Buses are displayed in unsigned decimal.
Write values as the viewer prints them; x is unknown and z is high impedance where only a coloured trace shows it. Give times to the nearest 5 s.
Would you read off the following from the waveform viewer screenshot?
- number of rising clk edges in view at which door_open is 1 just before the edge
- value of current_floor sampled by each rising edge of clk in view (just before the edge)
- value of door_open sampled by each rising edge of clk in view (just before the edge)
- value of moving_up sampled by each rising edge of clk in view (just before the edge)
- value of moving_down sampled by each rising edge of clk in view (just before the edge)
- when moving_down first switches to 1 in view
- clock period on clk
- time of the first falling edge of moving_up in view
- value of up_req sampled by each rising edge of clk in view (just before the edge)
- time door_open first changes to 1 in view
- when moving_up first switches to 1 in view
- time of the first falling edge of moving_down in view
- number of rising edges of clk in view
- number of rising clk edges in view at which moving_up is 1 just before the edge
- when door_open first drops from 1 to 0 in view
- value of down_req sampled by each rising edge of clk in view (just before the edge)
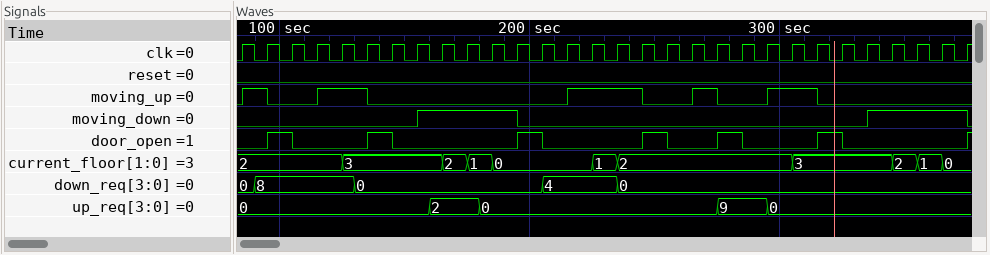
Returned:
6
2, 2, 2, 2, 2, 3, 3, 3, 3, 2, 1, 0, 0, 0, 0, 1, 2, 2, 2, 2, 2, 2, 2, 3, 3, 3, 3, 2, 1, 0
0 0 1 0 0 0 1 0 0 0 0 0 1 0 0 0 0 1 0 0 1 0 0 0 1 0 0 0 0 0
0 1 0 0 1 1 0 0 0 0 0 0 0 0 1 1 1 0 0 1 0 0 1 1 0 0 0 0 0 0
0 0 0 0 0 0 0 0 1 1 1 1 0 0 0 0 0 0 0 0 0 0 0 0 0 0 1 1 1 1
155 s
10 s
95 s
0, 0, 0, 0, 0, 0, 0, 0, 2, 2, 0, 0, 0, 0, 0, 0, 0, 0, 0, 0, 9, 9, 0, 0, 0, 0, 0, 0, 0, 0
95 s
85 s
195 s
30
9
105 s
0, 8, 8, 8, 8, 0, 0, 0, 0, 0, 0, 0, 0, 4, 4, 4, 0, 0, 0, 0, 0, 0, 0, 0, 0, 0, 0, 0, 0, 0
